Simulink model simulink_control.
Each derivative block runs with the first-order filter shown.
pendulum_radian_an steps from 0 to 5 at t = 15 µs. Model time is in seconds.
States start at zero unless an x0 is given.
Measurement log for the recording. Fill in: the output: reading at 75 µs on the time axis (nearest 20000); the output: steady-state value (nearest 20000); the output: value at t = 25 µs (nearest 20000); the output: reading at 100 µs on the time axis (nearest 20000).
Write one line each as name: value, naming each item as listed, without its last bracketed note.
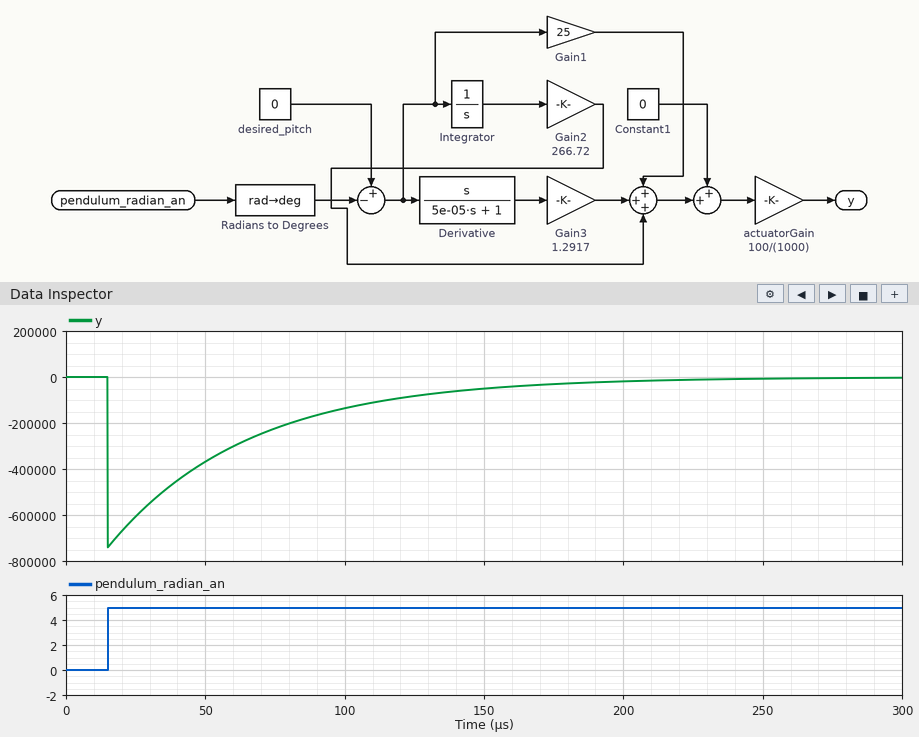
the output: reading at 75 µs on the time axis: -220000
the output: steady-state value: 0
the output: value at t = 25 µs: -600000
the output: reading at 100 µs on the time axis: -140000
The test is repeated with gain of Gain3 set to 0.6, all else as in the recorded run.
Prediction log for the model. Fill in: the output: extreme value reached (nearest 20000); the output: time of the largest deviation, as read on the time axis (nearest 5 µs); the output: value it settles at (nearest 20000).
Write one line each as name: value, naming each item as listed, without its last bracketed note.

the output: extreme value reached: -340000
the output: time of the largest deviation, as read on the time axis: 15 µs
the output: value it settles at: 0
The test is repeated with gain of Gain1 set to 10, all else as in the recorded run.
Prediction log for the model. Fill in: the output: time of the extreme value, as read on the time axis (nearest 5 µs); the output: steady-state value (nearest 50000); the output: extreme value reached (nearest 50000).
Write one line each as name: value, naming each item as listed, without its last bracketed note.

the output: time of the extreme value, as read on the time axis: 15 µs
the output: steady-state value: 0
the output: extreme value reached: -750000
